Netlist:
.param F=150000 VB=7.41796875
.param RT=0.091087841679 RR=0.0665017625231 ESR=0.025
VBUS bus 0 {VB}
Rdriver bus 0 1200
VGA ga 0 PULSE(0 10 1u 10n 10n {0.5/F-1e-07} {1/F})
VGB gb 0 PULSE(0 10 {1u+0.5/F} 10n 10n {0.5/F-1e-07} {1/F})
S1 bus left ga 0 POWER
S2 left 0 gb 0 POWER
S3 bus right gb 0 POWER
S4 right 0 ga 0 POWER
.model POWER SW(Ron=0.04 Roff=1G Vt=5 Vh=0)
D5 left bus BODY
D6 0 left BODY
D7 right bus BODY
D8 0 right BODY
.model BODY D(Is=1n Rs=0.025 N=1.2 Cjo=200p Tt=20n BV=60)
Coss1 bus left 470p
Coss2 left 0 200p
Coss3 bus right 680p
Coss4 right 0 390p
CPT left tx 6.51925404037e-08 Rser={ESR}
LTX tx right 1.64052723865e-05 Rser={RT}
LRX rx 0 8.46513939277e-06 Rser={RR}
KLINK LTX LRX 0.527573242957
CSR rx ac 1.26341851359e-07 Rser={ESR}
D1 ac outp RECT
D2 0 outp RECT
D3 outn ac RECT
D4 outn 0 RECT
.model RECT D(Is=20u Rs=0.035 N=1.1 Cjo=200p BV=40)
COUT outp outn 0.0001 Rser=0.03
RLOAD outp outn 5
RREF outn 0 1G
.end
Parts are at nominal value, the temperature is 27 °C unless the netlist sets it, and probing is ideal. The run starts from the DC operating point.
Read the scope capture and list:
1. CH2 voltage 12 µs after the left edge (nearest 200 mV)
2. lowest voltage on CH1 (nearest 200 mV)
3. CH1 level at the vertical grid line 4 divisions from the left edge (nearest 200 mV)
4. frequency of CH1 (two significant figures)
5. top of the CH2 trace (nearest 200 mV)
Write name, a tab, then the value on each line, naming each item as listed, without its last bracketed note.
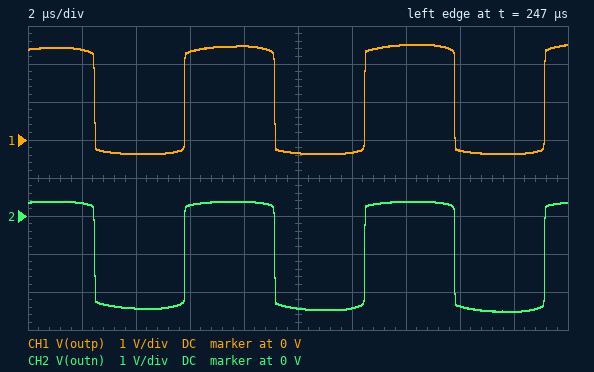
CH2 voltage 12 µs after the left edge	-2.4 V
lowest voltage on CH1	-400 mV
CH1 level at the vertical grid line 4 divisions from the left edge	2.4 V
frequency of CH1	150 kHz
top of the CH2 trace	400 mV
